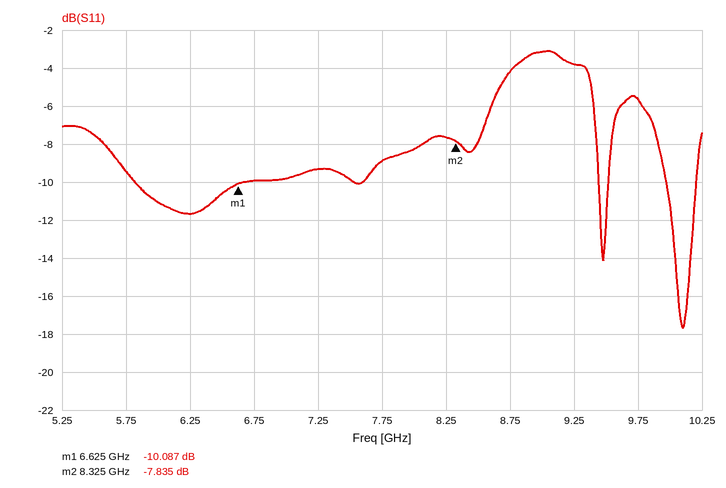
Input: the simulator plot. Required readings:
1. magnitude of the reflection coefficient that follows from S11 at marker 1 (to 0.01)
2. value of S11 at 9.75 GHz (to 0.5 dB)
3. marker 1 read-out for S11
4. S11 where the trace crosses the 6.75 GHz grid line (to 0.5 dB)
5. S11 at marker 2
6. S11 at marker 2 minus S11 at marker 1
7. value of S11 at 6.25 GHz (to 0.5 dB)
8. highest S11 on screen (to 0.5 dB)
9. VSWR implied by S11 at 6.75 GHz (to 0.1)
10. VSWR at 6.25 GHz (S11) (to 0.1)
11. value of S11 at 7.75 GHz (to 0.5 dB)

0.31
-5.5 dB
-10.087 dB
-10.0 dB
-7.835 dB
2.252 dB
-11.5 dB
-3.0 dB
1.9
1.7
-9.0 dB
